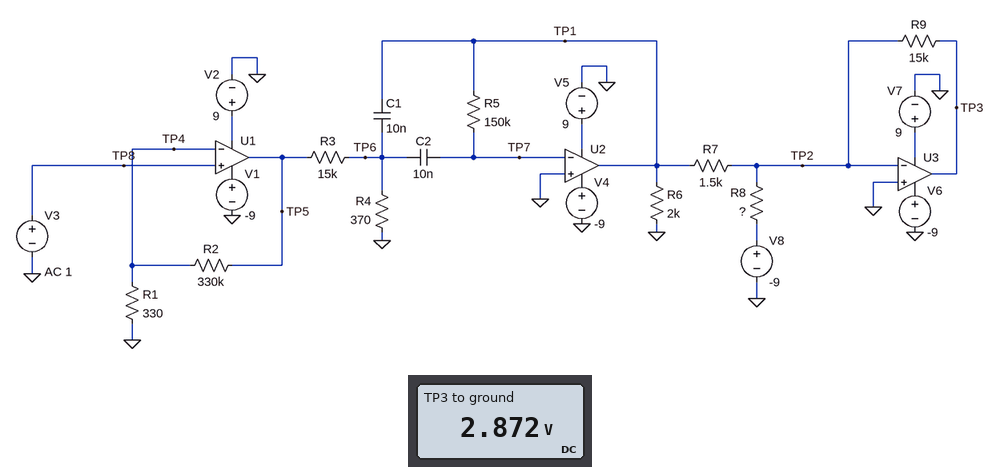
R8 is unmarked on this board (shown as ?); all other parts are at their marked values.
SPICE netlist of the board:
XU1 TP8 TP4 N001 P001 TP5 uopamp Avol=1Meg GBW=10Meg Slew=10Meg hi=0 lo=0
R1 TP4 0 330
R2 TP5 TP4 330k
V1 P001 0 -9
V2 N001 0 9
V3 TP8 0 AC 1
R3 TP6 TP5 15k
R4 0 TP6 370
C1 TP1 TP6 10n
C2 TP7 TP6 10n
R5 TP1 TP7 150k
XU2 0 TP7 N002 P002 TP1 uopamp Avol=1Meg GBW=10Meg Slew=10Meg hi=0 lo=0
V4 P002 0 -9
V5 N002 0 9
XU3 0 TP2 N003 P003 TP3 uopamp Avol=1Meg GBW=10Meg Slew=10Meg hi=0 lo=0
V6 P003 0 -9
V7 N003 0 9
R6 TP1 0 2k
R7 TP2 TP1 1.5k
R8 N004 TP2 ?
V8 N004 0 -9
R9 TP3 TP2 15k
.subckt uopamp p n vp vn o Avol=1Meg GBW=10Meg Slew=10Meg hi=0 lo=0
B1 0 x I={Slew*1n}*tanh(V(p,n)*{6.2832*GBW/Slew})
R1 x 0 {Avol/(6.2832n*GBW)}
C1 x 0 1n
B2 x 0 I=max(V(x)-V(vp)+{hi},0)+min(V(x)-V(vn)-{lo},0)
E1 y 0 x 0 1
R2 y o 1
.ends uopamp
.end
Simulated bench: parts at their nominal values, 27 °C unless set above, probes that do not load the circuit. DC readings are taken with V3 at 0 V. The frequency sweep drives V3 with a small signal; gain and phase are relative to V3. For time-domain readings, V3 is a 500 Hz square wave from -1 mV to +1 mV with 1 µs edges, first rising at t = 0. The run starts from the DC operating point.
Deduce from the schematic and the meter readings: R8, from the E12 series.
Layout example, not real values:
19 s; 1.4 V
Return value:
47 kΩ
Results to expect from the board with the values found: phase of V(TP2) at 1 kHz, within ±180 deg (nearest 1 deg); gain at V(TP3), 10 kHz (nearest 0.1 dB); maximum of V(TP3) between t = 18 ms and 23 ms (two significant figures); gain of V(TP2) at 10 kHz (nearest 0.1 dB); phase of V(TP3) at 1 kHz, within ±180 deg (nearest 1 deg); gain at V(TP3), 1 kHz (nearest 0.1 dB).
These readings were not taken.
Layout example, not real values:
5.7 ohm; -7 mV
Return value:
-10 deg; 57.9 dB; 9.0 V; -2.1 dB; 81 deg; 69.2 dB
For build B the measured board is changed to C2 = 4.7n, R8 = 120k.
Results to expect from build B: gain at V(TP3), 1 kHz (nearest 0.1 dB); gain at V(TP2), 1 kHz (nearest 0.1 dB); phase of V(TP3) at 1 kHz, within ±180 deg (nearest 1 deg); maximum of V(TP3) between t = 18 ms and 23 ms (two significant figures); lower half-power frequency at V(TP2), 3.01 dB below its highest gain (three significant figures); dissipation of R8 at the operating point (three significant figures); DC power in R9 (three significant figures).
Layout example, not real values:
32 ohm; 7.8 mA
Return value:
61.4 dB; -18.6 dB; 82 deg; 5.8 V; 3.00 kHz; 675 µW; 84.4 µW
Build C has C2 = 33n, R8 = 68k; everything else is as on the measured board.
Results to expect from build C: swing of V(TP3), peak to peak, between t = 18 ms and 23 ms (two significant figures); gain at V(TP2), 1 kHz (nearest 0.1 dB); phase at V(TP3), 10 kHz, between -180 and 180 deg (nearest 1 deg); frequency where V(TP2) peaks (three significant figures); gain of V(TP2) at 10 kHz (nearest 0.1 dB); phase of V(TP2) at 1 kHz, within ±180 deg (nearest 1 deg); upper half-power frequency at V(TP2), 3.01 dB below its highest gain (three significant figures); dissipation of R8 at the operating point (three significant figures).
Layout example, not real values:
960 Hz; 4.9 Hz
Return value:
18 V; 7.7 dB; -135 deg; 1.19 kHz; -2.4 dB; -25 deg; 1.27 kHz; 1.19 mW
